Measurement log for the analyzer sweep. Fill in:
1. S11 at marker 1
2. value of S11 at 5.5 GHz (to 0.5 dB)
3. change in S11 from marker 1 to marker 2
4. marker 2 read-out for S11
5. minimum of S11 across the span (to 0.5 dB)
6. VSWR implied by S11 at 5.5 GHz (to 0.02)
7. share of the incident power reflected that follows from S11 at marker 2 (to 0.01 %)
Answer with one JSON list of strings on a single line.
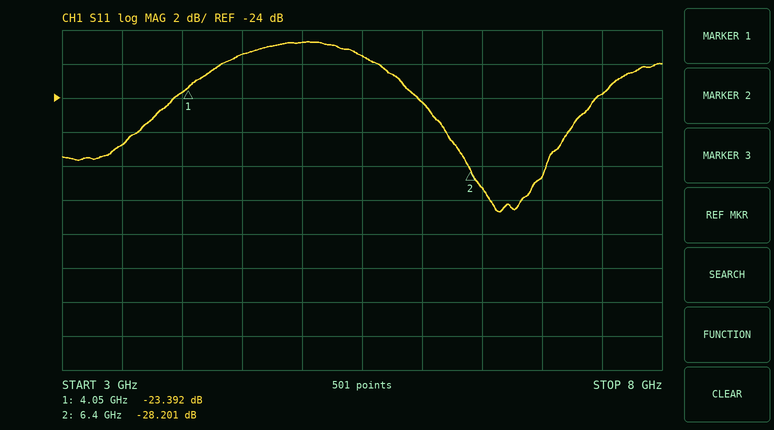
["-23.392 dB", "-21.5 dB", "-4.809 dB", "-28.201 dB", "-30.5 dB", "1.18", "0.15 %"]
